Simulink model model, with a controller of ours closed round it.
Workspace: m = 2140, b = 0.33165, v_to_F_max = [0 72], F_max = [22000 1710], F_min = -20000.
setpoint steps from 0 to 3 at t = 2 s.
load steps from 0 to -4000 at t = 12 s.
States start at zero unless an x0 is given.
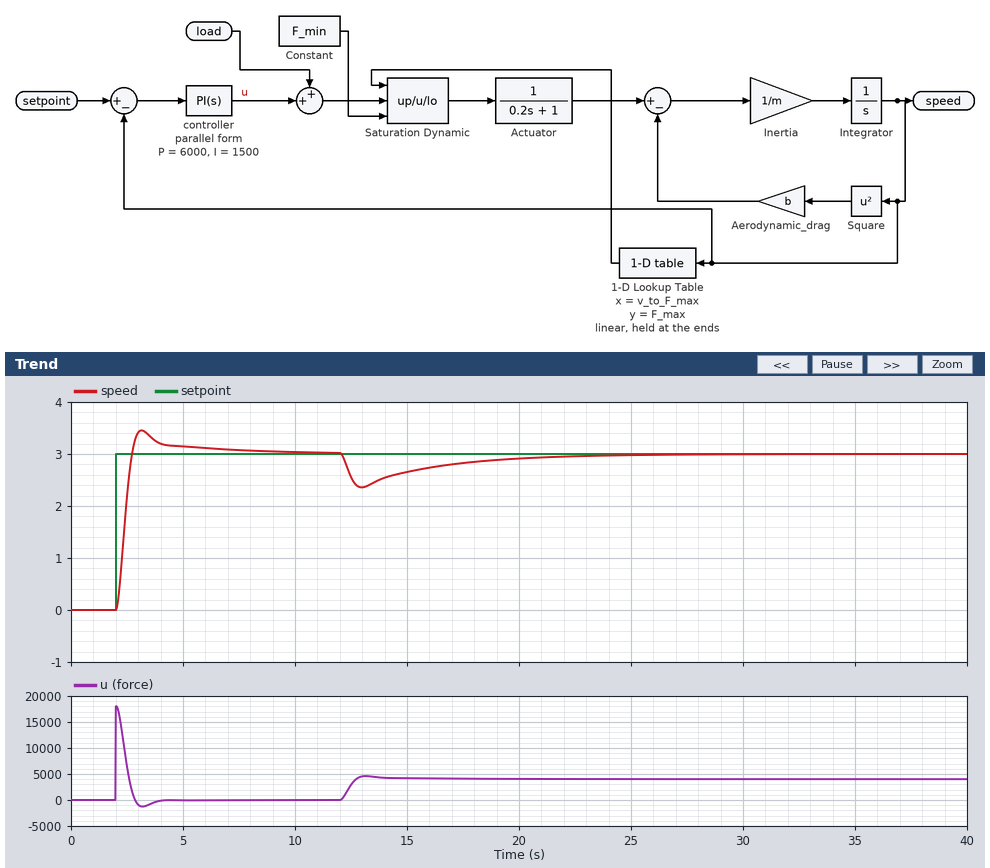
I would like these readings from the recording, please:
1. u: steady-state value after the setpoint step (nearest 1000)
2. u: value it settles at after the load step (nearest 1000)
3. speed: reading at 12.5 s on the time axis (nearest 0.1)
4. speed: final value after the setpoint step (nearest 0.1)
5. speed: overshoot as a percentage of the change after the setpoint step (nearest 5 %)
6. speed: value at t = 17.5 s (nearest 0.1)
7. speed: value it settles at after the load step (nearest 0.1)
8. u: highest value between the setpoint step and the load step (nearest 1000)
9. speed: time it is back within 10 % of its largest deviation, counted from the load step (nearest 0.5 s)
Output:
0
4000
2.6
3.0
15 %
2.8
3.0
18000
9.0 s
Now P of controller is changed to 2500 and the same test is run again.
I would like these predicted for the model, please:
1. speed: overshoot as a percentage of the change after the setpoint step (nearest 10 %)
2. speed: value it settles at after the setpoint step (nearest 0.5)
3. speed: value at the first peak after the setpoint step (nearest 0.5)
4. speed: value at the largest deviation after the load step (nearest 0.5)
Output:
30 %
3.0
4.0
2.0
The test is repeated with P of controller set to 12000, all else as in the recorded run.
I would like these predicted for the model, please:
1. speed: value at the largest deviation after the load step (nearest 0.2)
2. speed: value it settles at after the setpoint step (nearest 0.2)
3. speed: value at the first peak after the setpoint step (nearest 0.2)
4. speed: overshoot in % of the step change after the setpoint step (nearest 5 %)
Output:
2.6
3.0
3.6
20 %
